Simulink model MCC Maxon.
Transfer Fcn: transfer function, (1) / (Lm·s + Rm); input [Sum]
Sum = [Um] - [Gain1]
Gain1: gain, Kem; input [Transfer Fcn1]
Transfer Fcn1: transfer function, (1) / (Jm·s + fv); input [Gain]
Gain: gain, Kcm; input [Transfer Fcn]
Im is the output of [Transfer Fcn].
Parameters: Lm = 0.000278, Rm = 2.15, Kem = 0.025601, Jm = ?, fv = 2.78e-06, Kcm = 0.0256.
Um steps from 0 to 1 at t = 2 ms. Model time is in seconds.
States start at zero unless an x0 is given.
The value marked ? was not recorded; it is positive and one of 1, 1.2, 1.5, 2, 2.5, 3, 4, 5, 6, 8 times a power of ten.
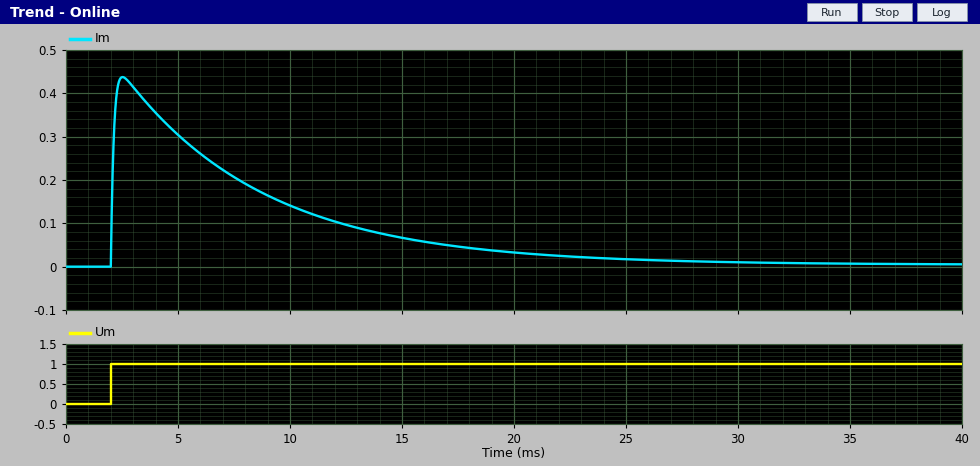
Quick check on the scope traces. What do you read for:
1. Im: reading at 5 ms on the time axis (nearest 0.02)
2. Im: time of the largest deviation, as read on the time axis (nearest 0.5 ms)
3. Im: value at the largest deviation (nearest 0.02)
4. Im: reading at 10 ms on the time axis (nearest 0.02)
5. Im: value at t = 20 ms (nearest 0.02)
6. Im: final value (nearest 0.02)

0.30
2.5 ms
0.44
0.14
0.04
0.00
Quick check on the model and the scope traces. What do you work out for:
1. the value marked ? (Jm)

2e-06
